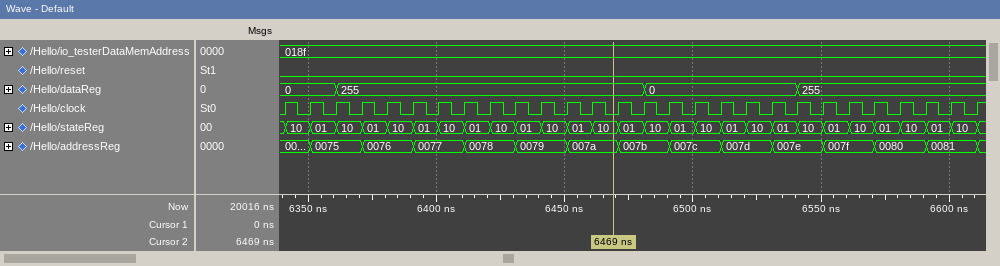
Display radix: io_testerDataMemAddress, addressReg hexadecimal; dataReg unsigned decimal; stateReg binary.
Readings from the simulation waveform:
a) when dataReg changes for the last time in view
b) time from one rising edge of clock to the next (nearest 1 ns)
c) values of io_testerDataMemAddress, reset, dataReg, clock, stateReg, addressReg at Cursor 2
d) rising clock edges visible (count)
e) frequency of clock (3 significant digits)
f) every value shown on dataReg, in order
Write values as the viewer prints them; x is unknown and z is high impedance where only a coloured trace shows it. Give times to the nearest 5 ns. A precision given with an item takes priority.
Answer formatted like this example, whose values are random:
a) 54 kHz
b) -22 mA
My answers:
a) 6540 ns
b) 10 ns
c) io_testerDataMemAddress=018f, reset=0, dataReg=255, clock=0, stateReg=10, addressReg=007a
d) 28
e) 100 MHz
f) 0, 255, 0, 255
